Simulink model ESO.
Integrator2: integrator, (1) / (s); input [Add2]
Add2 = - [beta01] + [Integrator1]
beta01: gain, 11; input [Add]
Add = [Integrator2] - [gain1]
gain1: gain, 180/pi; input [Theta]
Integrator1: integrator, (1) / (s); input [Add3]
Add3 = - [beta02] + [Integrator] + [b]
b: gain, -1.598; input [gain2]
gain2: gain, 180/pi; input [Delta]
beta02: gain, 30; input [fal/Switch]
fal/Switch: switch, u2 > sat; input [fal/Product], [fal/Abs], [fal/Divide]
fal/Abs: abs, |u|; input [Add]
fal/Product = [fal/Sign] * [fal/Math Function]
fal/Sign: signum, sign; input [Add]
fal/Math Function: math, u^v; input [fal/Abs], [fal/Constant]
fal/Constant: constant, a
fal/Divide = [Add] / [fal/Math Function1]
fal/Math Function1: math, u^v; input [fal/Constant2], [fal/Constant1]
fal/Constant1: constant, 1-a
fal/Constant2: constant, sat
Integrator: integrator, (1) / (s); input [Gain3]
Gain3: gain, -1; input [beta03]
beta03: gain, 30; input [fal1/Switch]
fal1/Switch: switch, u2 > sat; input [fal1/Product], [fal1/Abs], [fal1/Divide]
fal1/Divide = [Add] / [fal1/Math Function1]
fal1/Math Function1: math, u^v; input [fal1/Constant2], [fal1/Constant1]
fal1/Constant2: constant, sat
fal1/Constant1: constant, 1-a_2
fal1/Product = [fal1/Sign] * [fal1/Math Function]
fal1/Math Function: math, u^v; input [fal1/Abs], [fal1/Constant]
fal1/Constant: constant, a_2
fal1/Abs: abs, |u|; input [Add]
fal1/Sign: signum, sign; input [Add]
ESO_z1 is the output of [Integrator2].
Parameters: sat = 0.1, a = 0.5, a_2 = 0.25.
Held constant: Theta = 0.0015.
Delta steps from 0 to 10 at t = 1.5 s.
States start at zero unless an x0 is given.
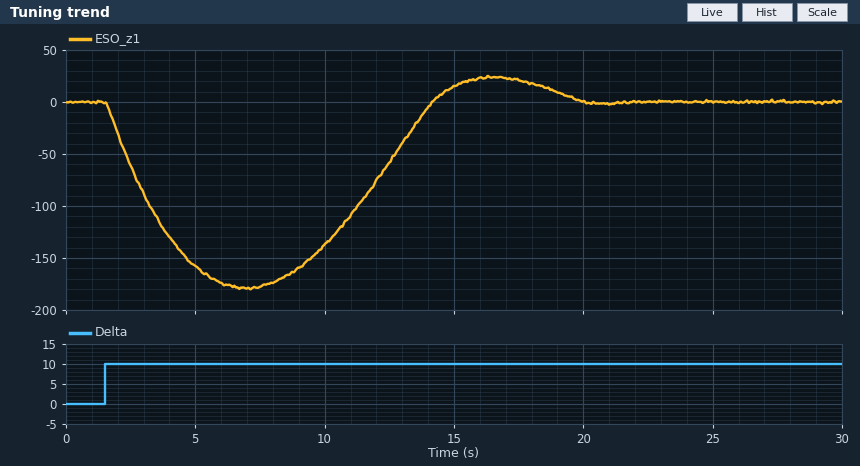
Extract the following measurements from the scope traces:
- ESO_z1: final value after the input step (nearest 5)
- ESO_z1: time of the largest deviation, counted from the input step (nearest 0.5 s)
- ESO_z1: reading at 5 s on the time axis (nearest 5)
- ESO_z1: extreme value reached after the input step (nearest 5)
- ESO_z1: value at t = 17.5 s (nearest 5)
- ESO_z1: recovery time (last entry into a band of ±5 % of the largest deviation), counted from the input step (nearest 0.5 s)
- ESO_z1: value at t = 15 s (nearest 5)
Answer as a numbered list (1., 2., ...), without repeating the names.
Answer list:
1. 0
2. 5.5 s
3. -160
4. -180
5. 20
6. 17.5 s
7. 15
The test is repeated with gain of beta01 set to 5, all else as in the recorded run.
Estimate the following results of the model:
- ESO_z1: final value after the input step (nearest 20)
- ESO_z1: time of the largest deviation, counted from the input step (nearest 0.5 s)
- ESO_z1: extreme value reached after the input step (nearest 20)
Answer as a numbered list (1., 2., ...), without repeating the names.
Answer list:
1. 0
2. 4.0 s
3. -280
